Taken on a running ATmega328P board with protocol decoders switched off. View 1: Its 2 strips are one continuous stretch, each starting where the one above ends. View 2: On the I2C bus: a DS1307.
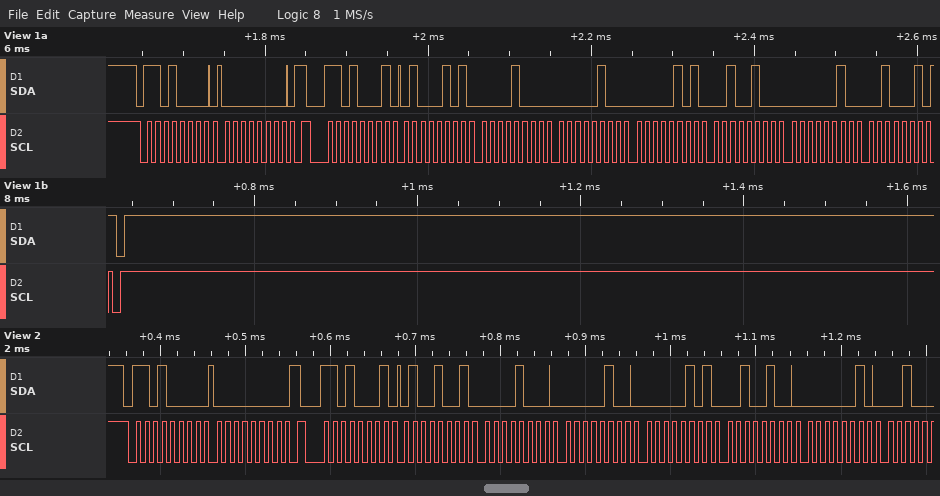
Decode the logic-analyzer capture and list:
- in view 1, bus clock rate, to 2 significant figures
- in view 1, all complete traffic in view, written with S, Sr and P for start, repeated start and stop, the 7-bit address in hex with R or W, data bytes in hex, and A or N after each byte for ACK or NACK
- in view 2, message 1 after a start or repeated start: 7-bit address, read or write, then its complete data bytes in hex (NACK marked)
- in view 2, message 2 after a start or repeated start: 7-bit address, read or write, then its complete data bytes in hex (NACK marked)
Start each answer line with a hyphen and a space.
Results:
- 100 kHz
- S 68W A 00 A Sr 68R A 45 A 08 A 04 A 05 A 24 A 02 A 22 N P
- 0x68 write: 00
- 0x68 read: 49 08 04 05 24 02
